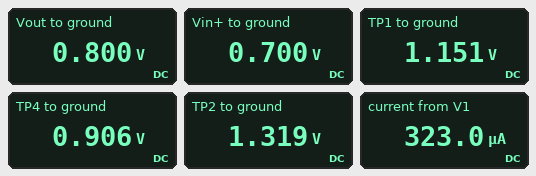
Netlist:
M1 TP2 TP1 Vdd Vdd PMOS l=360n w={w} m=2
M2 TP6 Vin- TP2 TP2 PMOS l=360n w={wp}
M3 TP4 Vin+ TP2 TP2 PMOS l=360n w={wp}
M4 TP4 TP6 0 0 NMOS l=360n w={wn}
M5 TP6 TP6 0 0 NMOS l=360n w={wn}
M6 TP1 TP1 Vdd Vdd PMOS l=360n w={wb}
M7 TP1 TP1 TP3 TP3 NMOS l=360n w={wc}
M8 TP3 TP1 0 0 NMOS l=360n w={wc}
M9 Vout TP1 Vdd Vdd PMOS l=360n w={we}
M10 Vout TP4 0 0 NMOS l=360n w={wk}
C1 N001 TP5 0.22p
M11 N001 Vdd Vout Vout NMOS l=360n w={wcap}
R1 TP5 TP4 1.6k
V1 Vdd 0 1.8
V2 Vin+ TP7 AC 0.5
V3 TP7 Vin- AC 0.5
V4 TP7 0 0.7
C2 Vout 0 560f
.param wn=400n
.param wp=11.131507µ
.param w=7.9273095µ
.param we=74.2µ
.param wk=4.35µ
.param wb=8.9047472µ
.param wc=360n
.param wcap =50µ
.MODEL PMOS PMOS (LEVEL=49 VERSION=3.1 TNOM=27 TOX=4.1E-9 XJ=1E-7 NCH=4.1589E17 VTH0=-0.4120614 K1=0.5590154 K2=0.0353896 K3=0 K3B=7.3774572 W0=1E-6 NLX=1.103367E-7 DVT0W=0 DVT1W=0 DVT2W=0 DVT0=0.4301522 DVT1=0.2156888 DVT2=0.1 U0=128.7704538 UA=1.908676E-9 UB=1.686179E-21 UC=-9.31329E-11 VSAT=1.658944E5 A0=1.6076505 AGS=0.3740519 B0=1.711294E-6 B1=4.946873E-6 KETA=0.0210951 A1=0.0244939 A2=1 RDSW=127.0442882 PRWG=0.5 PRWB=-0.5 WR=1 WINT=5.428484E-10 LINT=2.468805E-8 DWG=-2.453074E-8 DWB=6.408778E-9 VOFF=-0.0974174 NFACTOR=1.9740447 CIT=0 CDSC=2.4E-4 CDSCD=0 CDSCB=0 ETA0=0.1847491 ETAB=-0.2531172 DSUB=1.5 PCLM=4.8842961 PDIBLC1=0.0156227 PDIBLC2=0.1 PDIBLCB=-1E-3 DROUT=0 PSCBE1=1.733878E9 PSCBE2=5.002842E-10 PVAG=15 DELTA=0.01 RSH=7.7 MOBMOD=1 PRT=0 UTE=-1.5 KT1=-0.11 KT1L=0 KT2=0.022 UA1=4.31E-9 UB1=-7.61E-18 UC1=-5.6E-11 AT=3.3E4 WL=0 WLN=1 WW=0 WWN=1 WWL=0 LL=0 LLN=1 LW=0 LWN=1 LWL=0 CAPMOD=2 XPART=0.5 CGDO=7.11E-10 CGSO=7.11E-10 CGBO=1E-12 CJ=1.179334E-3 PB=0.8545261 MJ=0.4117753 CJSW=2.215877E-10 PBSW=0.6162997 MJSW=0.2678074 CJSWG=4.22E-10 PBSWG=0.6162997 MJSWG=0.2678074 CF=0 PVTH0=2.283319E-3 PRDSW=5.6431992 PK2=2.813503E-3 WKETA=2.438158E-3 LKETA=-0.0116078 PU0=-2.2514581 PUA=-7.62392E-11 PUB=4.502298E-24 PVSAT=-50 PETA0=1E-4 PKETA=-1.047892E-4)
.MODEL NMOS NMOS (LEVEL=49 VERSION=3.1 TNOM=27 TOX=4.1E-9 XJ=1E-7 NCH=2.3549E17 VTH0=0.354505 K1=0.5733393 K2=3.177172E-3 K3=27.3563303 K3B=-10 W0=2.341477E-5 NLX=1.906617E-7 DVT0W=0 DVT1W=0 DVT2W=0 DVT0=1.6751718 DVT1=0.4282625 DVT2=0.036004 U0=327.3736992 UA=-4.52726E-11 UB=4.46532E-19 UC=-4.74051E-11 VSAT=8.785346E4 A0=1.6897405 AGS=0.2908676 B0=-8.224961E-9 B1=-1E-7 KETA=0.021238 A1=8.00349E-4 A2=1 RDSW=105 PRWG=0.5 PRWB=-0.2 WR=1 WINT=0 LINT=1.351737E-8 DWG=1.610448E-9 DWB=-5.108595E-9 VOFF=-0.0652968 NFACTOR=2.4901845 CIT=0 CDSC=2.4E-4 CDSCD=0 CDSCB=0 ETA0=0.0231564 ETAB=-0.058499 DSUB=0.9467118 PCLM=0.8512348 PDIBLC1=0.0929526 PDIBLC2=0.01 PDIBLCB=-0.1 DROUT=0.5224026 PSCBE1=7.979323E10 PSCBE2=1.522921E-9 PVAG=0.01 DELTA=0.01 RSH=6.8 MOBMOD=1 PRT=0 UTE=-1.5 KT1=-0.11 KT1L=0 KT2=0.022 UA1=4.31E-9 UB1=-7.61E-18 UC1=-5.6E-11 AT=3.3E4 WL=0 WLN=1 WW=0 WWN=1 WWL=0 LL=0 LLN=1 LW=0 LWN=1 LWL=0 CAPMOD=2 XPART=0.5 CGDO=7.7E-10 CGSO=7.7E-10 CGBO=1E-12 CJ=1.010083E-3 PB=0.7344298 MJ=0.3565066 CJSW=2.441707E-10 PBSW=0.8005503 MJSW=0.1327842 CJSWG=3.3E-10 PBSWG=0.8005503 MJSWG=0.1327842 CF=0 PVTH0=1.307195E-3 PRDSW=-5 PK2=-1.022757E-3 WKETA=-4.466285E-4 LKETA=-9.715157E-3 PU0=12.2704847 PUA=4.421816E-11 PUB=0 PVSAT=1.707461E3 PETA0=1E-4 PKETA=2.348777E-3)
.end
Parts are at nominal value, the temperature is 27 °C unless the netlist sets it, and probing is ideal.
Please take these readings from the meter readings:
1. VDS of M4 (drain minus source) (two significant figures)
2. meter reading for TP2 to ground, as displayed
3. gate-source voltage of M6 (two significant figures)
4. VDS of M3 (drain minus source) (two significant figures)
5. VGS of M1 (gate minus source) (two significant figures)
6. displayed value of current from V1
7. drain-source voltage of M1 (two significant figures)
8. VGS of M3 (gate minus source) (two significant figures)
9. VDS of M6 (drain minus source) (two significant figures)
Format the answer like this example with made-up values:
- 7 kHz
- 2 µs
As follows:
- 910 mV
- 1.319 V
- -650 mV
- -410 mV
- -650 mV
- 323.0 µA
- -480 mV
- -620 mV
- -650 mV
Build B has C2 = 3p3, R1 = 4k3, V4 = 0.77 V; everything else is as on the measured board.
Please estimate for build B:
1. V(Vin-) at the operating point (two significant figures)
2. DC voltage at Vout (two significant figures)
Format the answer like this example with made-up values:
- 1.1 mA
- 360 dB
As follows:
- 770 mV
- 840 mV
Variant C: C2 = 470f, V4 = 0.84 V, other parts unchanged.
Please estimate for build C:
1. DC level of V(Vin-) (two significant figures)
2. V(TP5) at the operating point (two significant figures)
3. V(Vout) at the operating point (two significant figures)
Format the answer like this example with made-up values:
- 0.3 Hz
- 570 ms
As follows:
- 840 mV
- 900 mV
- 890 mV
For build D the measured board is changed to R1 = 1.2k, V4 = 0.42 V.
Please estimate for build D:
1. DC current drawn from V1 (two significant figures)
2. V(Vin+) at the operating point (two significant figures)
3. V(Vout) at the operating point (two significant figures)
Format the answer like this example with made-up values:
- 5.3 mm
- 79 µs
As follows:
- 330 µA
- 420 mV
- 650 mV
